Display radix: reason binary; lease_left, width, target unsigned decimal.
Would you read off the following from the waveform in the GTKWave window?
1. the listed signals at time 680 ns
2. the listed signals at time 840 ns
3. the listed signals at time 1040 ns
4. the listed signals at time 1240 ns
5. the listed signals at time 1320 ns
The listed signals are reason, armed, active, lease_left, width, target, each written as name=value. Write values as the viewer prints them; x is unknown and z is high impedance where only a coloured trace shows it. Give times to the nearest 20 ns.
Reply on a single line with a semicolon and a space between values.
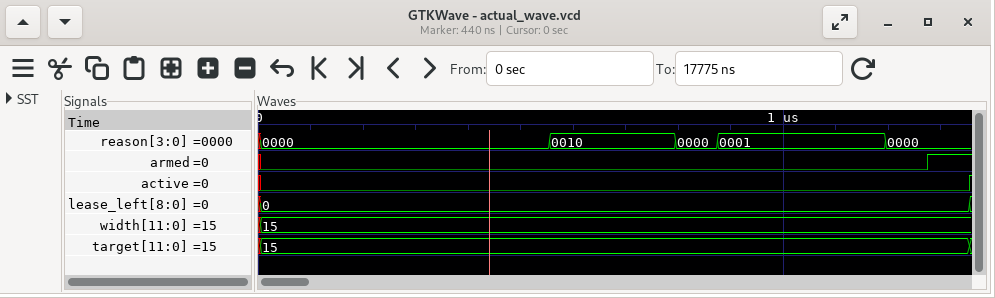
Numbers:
reason=0010, armed=0, active=0, lease_left=0, width=15, target=15; reason=0000, armed=0, active=0, lease_left=0, width=15, target=15; reason=0001, armed=0, active=0, lease_left=0, width=15, target=15; reason=0000, armed=0, active=0, lease_left=0, width=15, target=15; reason=0000, armed=1, active=0, lease_left=0, width=15, target=15
